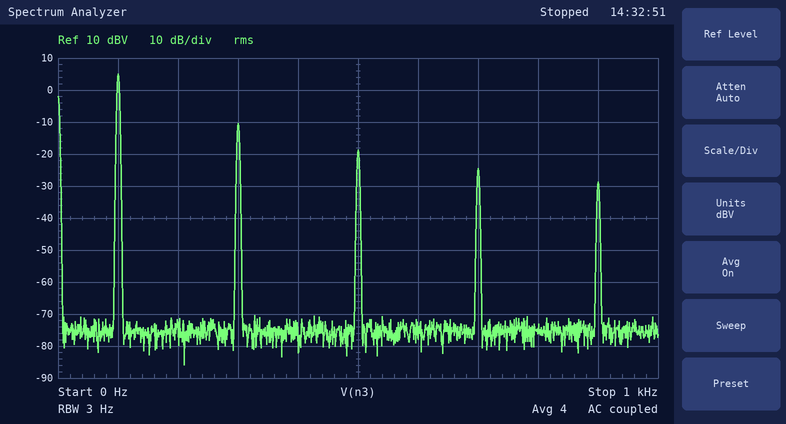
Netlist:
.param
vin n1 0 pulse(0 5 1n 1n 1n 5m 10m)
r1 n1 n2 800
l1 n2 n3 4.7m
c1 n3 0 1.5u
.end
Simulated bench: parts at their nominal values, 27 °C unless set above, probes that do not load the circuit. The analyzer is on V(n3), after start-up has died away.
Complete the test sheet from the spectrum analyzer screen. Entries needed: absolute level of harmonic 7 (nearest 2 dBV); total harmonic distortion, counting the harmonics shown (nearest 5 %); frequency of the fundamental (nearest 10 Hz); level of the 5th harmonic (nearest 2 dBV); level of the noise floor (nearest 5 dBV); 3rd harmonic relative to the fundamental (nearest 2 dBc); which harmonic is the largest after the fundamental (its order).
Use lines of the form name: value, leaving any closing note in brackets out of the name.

absolute level of harmonic 7: -24 dBV
total harmonic distortion, counting the harmonics shown: 20 %
frequency of the fundamental: 100 Hz
level of the 5th harmonic: -18 dBV
level of the noise floor: -75 dBV
3rd harmonic relative to the fundamental: -16 dBc
which harmonic is the largest after the fundamental: 3
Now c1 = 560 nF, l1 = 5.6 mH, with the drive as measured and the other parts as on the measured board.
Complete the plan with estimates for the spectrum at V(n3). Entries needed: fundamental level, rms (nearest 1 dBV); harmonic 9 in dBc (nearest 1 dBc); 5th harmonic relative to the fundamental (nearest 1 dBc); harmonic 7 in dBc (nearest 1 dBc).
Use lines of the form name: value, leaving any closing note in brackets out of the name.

fundamental level, rms: 7 dBV
harmonic 9 in dBc: -27 dBc
5th harmonic relative to the fundamental: -18 dBc
harmonic 7 in dBc: -23 dBc
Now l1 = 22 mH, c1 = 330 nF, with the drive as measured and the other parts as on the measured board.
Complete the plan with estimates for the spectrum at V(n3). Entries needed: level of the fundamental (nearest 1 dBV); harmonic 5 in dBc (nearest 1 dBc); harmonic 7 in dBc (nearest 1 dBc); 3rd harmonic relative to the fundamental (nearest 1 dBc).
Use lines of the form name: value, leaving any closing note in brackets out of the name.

level of the fundamental: 7 dBV
harmonic 5 in dBc: -16 dBc
harmonic 7 in dBc: -20 dBc
3rd harmonic relative to the fundamental: -10 dBc
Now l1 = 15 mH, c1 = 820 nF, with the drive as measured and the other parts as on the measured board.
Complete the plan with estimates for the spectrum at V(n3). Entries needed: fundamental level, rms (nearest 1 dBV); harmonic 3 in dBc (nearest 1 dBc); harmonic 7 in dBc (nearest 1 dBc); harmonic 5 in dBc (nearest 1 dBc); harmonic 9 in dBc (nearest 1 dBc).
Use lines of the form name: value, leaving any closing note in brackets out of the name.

fundamental level, rms: 6 dBV
harmonic 3 in dBc: -13 dBc
harmonic 7 in dBc: -26 dBc
harmonic 5 in dBc: -20 dBc
harmonic 9 in dBc: -30 dBc
